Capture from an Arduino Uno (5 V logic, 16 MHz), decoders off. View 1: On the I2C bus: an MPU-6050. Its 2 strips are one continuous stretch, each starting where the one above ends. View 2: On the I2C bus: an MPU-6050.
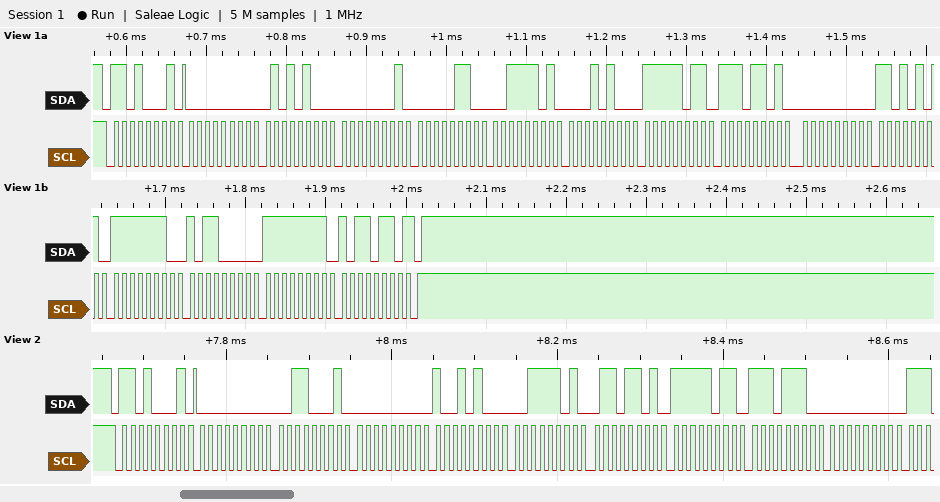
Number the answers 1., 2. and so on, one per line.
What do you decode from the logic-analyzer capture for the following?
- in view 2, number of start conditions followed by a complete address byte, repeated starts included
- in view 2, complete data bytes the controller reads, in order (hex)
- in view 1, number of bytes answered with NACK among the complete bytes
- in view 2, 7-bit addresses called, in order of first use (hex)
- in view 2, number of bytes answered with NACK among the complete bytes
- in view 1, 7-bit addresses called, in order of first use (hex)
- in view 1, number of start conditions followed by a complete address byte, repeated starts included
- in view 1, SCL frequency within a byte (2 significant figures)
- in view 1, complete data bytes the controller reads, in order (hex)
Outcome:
1. 1
2. 00 31 00 94 3D 6D FB EE 00
3. 1
4. 0x68
5. 0
6. 0x68
7. 1
8. 100 kHz
9. 00 54 01 06 3D 14 FB ED 00 D5 FE B0 FF B6
